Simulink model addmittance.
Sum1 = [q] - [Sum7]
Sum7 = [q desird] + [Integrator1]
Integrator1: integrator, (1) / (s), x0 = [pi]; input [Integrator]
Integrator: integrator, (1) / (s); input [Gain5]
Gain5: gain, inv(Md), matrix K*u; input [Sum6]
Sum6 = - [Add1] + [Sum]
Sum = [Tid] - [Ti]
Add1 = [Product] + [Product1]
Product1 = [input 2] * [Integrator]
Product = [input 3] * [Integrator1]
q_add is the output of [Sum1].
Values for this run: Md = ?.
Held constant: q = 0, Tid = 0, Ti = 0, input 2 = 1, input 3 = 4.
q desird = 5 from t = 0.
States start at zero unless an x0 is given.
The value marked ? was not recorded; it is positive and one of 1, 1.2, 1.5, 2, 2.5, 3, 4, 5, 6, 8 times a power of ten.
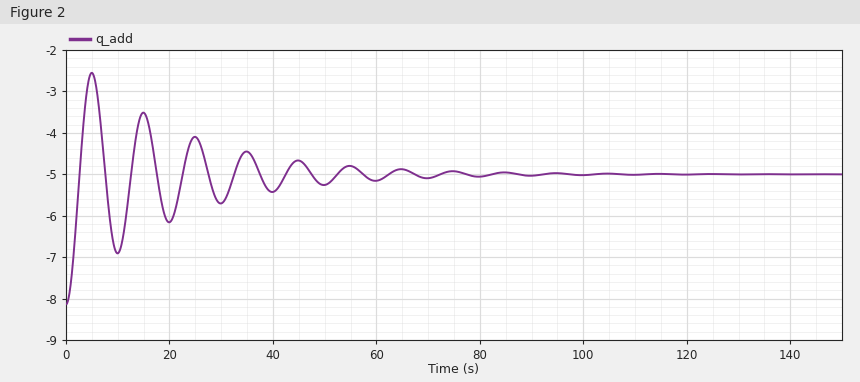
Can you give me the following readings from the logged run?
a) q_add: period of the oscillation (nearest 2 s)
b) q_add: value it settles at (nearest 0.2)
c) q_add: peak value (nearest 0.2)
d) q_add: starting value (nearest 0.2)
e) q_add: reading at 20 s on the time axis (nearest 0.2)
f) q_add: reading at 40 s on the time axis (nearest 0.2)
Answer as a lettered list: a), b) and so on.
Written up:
a) 10 s
b) -5.0
c) -2.6
d) -8.2
e) -6.2
f) -5.4
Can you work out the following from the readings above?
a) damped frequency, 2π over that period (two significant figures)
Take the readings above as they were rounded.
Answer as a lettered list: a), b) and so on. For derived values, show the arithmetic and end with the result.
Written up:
a) 2π / 10 = 0.63 rad/s
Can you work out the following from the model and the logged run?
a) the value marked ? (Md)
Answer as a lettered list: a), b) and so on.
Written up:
a) 10
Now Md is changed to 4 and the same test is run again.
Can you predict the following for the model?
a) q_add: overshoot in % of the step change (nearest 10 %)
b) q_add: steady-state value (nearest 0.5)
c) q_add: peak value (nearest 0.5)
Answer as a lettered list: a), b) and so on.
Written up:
a) 70 %
b) -5.0
c) -3.0
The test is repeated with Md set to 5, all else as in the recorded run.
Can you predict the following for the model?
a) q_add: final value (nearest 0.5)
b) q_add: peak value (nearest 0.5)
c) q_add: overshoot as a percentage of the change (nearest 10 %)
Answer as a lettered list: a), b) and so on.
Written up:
a) -5.0
b) -3.0
c) 70 %
